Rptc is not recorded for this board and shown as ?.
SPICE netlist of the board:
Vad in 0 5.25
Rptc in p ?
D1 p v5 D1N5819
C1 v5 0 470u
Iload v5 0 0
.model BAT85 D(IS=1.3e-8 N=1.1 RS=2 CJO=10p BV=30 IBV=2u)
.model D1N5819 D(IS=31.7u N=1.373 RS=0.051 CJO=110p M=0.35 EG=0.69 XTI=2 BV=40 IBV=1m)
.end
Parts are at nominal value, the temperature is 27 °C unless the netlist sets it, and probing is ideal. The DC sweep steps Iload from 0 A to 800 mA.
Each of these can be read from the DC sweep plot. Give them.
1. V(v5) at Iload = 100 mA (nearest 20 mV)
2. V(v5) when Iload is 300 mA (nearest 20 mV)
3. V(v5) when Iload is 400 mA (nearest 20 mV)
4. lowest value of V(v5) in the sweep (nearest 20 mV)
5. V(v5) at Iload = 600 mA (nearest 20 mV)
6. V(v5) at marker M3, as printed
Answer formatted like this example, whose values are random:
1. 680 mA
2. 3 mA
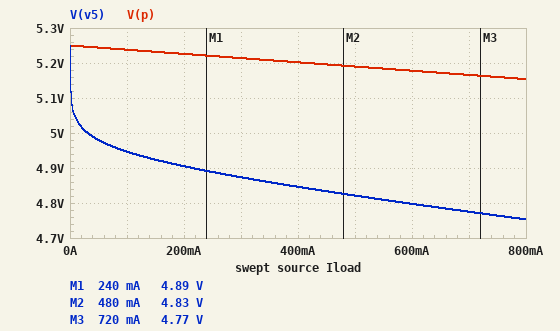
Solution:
1. 4.94 V
2. 4.88 V
3. 4.84 V
4. 4.76 V
5. 4.80 V
6. 4.77 V
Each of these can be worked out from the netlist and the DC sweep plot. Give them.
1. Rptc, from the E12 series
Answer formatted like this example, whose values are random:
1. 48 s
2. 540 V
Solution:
1. 0.12 Ω
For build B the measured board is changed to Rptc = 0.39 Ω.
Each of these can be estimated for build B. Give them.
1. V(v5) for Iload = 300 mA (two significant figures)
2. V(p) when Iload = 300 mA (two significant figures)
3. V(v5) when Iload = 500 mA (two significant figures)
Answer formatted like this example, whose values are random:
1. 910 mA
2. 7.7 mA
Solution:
1. 4.8 V
2. 5.1 V
3. 4.7 V
